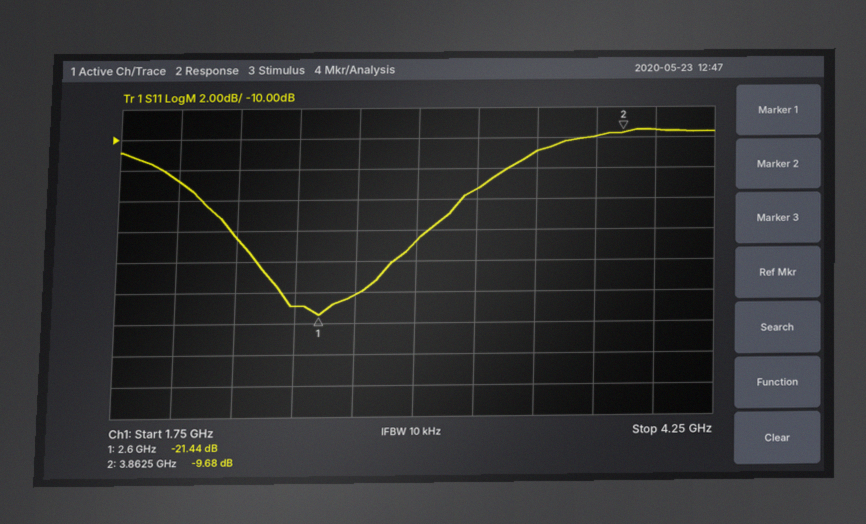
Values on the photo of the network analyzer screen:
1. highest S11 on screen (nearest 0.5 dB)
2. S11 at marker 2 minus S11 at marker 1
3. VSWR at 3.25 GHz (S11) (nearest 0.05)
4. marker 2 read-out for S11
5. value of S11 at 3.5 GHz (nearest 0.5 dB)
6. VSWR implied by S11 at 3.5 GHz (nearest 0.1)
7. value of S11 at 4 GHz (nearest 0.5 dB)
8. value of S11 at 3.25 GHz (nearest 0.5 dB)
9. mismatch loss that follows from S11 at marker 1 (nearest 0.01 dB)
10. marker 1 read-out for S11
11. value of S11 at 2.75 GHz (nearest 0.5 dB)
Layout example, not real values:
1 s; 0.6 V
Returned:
-9.5 dB; 11.76 dB; 1.55; -9.68 dB; -11.0 dB; 1.8; -9.5 dB; -13.5 dB; 0.03 dB; -21.44 dB; -20.0 dB
